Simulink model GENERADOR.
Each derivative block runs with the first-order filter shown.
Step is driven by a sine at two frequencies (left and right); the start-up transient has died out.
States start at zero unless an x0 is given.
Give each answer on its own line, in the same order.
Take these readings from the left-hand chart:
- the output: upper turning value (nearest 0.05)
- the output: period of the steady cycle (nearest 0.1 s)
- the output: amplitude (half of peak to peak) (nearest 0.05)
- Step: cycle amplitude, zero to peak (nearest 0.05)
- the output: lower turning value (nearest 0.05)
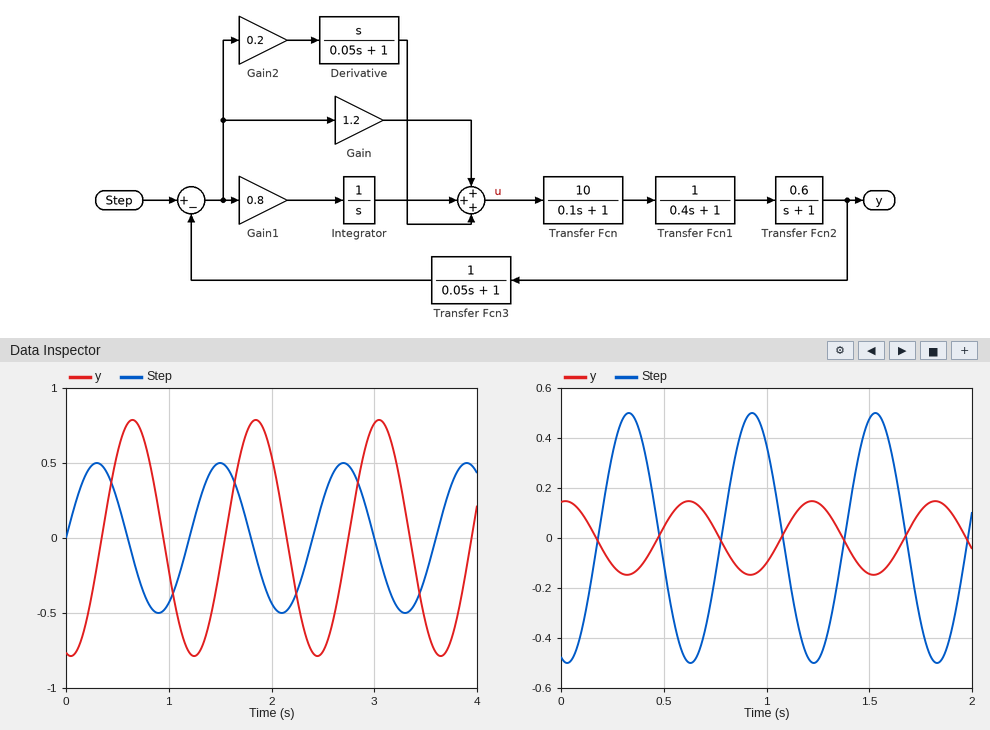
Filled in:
0.80
1.2 s
0.80
0.50
-0.80
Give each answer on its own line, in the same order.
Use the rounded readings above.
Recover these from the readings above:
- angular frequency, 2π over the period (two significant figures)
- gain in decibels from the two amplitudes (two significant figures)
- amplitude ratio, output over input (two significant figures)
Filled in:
5.2 rad/s
4.1 dB
1.6
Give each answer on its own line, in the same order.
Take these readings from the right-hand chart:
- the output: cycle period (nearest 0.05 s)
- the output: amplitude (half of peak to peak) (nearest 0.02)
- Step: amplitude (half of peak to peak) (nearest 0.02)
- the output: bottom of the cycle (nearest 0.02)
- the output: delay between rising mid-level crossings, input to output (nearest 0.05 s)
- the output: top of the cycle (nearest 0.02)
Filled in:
0.60 s
0.14
0.50
-0.14
0.30 s
0.14
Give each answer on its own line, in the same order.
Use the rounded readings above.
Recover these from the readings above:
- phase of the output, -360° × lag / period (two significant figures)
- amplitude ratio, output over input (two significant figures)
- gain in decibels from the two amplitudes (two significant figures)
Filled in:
-180°
0.28
-11 dB
